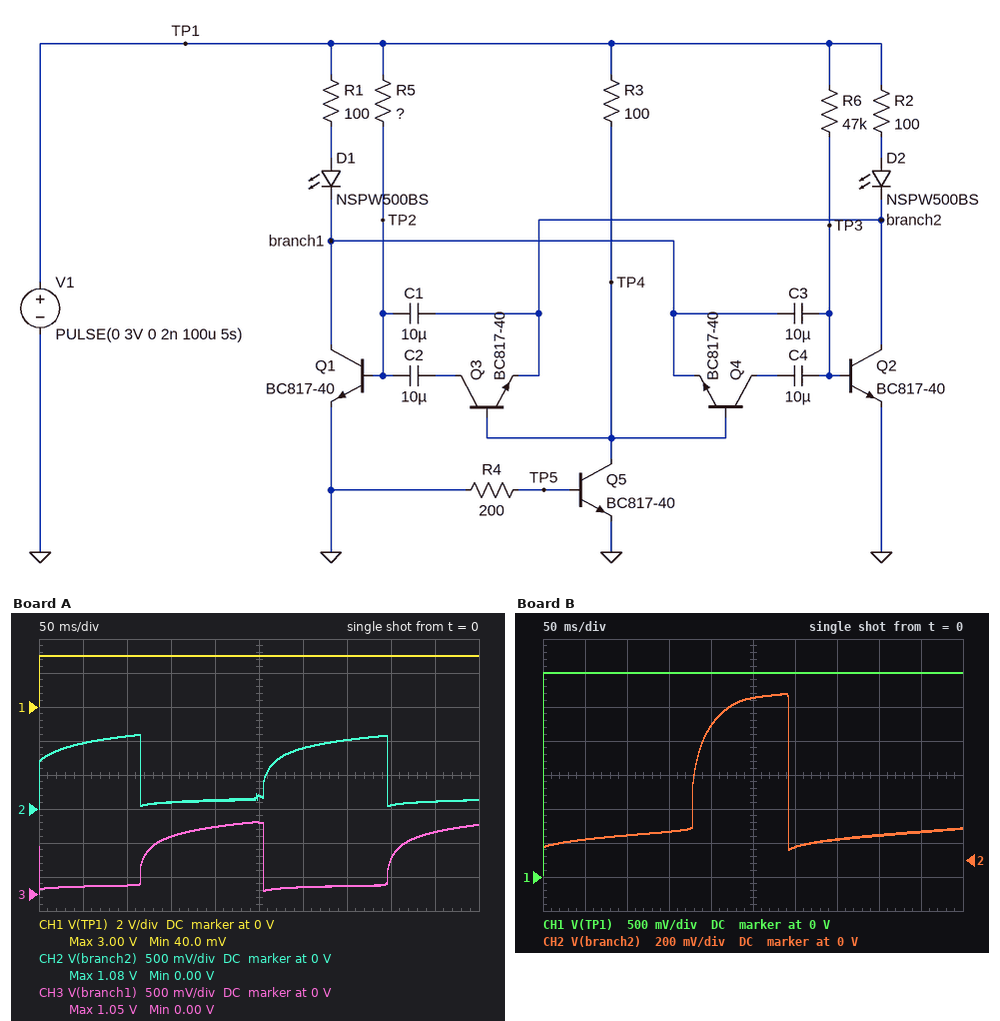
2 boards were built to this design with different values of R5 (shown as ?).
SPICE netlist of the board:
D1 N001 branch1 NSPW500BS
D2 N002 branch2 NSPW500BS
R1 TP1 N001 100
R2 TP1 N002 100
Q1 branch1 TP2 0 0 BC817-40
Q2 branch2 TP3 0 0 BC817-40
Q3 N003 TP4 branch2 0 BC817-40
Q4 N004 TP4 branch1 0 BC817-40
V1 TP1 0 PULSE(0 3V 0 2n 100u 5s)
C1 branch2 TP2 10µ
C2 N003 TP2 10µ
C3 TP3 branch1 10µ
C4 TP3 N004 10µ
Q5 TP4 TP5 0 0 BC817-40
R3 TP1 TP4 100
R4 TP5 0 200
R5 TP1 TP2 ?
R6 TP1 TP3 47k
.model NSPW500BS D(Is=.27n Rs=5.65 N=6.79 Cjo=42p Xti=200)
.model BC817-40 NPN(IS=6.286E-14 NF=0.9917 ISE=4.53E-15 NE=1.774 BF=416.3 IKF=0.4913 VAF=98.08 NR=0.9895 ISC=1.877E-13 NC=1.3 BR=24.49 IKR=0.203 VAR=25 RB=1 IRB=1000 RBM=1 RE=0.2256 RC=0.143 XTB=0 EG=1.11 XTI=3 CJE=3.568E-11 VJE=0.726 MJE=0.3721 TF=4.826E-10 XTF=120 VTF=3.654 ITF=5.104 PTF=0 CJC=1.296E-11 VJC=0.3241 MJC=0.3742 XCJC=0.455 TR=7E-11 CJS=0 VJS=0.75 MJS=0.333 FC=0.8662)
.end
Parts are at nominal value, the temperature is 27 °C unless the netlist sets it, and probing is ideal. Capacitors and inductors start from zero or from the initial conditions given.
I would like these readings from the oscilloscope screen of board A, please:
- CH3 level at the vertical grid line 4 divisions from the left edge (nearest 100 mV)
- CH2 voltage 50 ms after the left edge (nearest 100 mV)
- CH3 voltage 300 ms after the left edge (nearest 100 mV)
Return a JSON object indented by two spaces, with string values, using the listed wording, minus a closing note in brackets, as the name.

{
  "CH3 level at the vertical grid line 4 divisions from the left edge": "1.0 V",
  "CH2 voltage 50 ms after the left edge": "1.0 V",
  "CH3 voltage 300 ms after the left edge": "100 mV"
}
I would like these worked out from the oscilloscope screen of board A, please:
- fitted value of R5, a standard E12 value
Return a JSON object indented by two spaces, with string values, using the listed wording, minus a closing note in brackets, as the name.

{
  "fitted value of R5, a standard E12 value": "39 kΩ"
}
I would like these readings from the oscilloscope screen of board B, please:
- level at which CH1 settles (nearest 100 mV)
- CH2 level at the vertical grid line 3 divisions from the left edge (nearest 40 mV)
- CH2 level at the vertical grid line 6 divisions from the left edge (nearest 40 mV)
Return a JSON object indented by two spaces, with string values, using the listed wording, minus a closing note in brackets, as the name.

{
  "level at which CH1 settles": "3.0 V",
  "CH2 level at the vertical grid line 3 divisions from the left edge": "160 mV",
  "CH2 level at the vertical grid line 6 divisions from the left edge": "80 mV"
}
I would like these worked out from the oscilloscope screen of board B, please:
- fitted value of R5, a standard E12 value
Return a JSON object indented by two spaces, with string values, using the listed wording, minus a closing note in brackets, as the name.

{
  "fitted value of R5, a standard E12 value": "100 kΩ"
}
